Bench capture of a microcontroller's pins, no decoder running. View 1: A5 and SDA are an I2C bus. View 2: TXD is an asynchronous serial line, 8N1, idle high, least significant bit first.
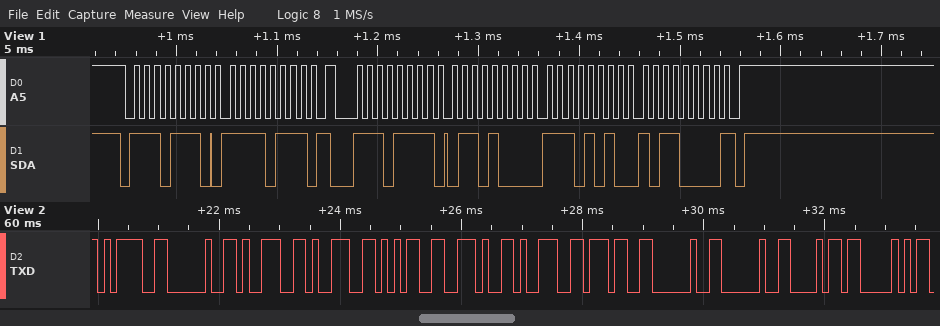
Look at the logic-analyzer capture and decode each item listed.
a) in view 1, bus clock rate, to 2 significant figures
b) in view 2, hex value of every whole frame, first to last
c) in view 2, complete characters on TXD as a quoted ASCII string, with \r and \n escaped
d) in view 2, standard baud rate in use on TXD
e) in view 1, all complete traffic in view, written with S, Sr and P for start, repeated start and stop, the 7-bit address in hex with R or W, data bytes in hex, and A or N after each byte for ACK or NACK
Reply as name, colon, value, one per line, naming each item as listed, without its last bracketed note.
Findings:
in view 1, bus clock rate, to 2 significant figures: 100 kHz
in view 2, hex value of every whole frame, first to last: 3D 20 39 39 35 2E 39 37 20 20 68 50
in view 2, complete characters on TXD as a quoted ASCII string, with \r and \n escaped: "= 995.97  hP"
in view 2, standard baud rate in use on TXD: 9600 baud
in view 1, all complete traffic in view, written with S, Sr and P for start, repeated start and stop, the 7-bit address in hex with R or W, data bytes in hex, and A or N after each byte for ACK or NACK: S 77W A F7 A Sr 77R A 68 A EA A B0 N P
